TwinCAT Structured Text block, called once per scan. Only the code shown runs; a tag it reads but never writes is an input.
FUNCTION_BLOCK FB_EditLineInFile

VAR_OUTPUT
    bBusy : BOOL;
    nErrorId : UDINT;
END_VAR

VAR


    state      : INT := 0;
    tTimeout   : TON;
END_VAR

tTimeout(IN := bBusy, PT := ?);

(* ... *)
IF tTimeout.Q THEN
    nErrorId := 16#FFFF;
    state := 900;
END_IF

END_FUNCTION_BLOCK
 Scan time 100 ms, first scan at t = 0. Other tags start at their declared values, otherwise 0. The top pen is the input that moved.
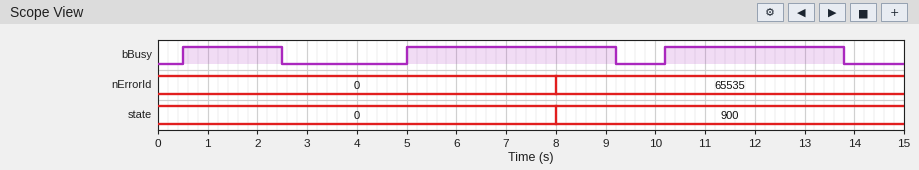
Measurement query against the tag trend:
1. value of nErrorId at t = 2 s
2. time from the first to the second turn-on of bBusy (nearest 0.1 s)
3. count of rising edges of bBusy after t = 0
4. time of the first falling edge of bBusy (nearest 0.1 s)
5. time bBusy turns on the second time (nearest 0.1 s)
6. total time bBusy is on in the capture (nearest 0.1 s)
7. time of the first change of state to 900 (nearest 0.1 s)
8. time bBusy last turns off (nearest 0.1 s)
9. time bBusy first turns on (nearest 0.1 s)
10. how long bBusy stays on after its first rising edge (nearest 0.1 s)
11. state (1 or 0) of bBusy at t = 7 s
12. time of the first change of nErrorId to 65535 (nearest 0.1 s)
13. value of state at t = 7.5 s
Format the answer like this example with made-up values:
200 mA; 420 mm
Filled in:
0; 4.5 s; 3; 2.5 s; 5.0 s; 9.8 s; 8.0 s; 13.8 s; 0.5 s; 2.0 s; 1; 8.0 s; 0
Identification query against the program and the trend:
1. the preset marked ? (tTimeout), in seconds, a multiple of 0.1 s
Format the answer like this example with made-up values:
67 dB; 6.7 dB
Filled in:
3.0 s
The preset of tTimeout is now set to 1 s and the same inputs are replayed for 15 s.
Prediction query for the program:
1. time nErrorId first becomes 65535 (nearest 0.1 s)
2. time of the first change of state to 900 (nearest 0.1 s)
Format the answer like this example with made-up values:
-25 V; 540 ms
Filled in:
1.5 s; 1.5 s
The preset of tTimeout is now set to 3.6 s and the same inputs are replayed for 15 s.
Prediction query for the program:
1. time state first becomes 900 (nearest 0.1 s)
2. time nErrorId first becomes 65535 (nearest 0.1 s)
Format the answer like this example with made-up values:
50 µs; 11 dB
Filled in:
8.6 s; 8.6 s
